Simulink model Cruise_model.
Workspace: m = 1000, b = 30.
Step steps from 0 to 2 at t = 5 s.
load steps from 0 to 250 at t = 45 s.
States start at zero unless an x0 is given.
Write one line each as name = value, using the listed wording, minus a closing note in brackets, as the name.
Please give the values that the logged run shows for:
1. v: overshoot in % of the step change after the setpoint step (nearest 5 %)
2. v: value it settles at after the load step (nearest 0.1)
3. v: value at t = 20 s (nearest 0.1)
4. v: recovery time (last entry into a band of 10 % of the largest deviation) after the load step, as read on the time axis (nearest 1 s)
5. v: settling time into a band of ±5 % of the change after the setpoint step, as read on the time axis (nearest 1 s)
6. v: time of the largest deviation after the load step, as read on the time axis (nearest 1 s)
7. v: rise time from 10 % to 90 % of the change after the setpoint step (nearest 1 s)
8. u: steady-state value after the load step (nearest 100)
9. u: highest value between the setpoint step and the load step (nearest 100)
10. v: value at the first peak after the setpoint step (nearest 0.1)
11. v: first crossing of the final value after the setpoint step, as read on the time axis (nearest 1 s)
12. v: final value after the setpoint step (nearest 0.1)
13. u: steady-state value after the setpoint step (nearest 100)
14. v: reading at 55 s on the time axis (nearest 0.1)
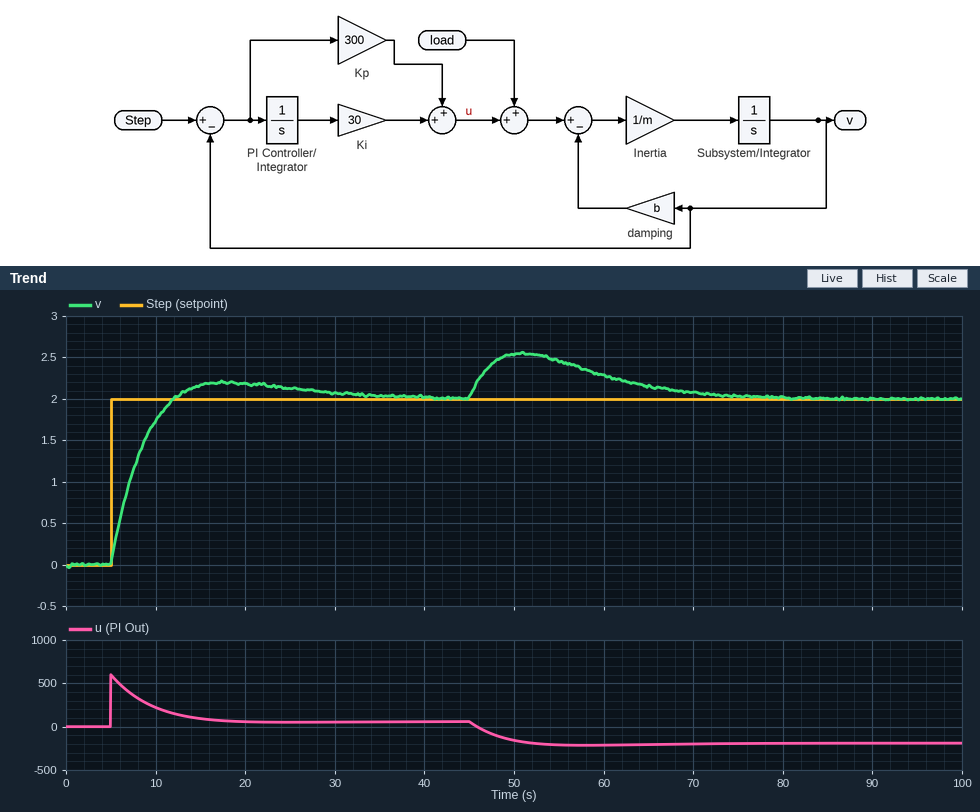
v: overshoot in % of the step change after the setpoint step = 10 %
v: value it settles at after the load step = 2.0
v: value at t = 20 s = 2.2
v: recovery time (last entry into a band of 10 % of the largest deviation) after the load step, as read on the time axis = 72 s
v: settling time into a band of ±5 % of the change after the setpoint step, as read on the time axis = 27 s
v: time of the largest deviation after the load step, as read on the time axis = 51 s
v: rise time from 10 % to 90 % of the change after the setpoint step = 5 s
u: steady-state value after the load step = -200
u: highest value between the setpoint step and the load step = 600
v: value at the first peak after the setpoint step = 2.2
v: first crossing of the final value after the setpoint step, as read on the time axis = 12 s
v: final value after the setpoint step = 2.0
u: steady-state value after the setpoint step = 100
v: reading at 55 s on the time axis = 2.5
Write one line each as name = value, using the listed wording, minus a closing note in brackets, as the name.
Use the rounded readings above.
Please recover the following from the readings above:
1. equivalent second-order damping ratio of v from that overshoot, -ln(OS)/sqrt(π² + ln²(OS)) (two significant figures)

equivalent second-order damping ratio of v from that overshoot, -ln(OS)/sqrt(π² + ln²(OS)) = 0.59
